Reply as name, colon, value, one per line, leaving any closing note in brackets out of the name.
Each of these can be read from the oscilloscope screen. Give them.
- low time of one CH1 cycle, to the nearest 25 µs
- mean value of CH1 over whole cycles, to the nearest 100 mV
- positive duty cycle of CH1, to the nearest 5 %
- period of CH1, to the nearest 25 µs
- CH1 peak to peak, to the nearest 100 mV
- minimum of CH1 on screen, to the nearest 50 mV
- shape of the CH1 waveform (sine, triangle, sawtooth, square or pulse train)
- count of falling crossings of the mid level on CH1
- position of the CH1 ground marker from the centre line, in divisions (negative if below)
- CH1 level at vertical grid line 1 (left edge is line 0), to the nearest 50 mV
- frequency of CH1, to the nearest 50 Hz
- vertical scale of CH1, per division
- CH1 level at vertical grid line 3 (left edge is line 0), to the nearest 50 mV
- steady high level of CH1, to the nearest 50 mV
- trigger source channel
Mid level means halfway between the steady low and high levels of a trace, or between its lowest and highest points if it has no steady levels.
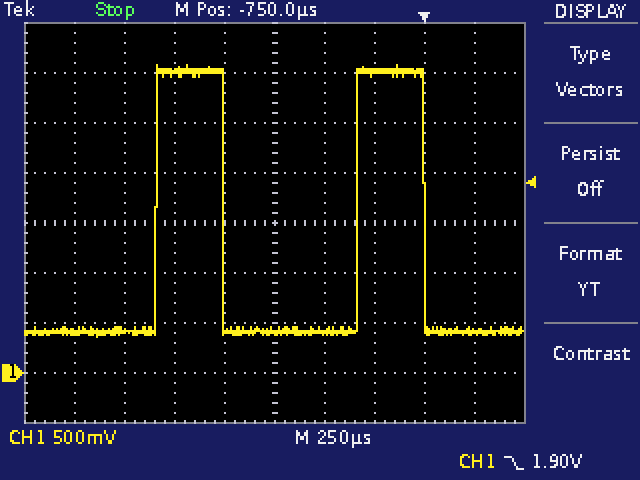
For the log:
low time of one CH1 cycle, to the nearest 25 µs: 675 µs
mean value of CH1 over whole cycles, to the nearest 100 mV: 1.3 V
positive duty cycle of CH1, to the nearest 5 %: 35 %
period of CH1, to the nearest 25 µs: 1.000 ms
CH1 peak to peak, to the nearest 100 mV: 2.70 V
minimum of CH1 on screen, to the nearest 50 mV: 350 mV
shape of the CH1 waveform: pulse train
count of falling crossings of the mid level on CH1: 2
position of the CH1 ground marker from the centre line, in divisions: -3.0 div
CH1 level at vertical grid line 1 (left edge is line 0), to the nearest 50 mV: 400 mV
frequency of CH1, to the nearest 50 Hz: 1.00 kHz
vertical scale of CH1, per division: 500 mV
CH1 level at vertical grid line 3 (left edge is line 0), to the nearest 50 mV: 3.00 V
steady high level of CH1, to the nearest 50 mV: 3.00 V
trigger source channel: CH1
